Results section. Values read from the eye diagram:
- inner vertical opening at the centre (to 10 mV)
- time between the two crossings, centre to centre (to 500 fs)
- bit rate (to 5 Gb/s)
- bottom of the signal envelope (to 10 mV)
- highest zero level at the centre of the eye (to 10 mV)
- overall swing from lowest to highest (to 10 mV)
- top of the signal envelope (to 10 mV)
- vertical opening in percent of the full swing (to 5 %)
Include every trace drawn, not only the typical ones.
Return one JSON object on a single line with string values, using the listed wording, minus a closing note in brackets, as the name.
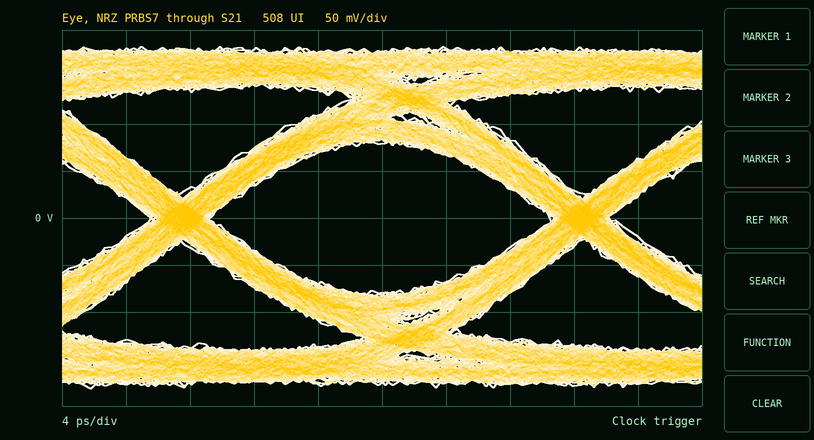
{"inner vertical opening at the centre": "160 mV", "time between the two crossings, centre to centre": "25.0 ps", "bit rate": "40 Gb/s", "bottom of the signal envelope": "-180 mV", "highest zero level at the centre of the eye": "-80 mV", "overall swing from lowest to highest": "360 mV", "top of the signal envelope": "180 mV", "vertical opening in percent of the full swing": "45 %"}
